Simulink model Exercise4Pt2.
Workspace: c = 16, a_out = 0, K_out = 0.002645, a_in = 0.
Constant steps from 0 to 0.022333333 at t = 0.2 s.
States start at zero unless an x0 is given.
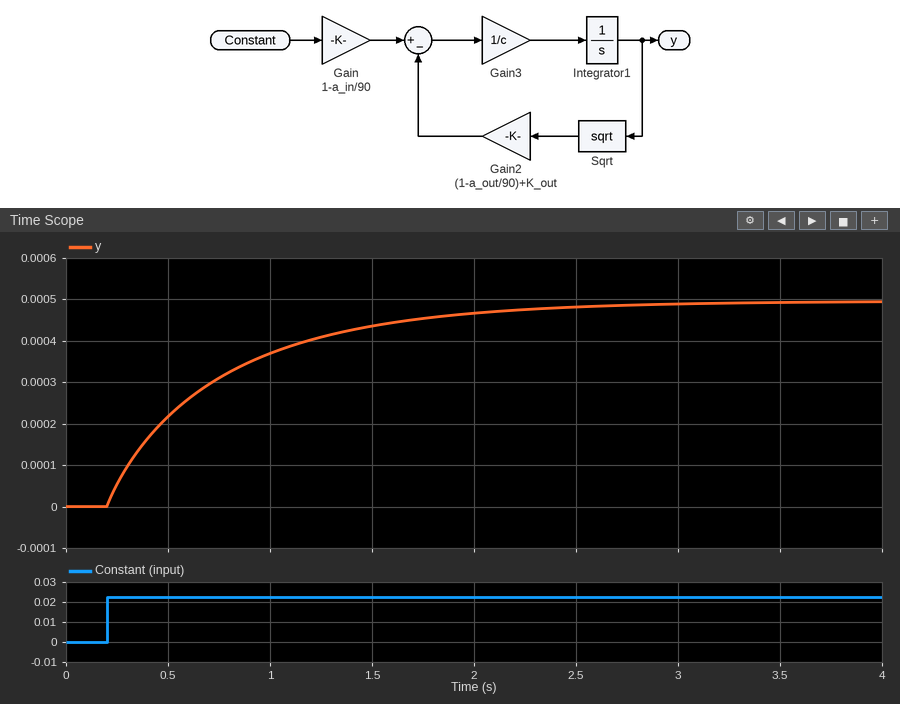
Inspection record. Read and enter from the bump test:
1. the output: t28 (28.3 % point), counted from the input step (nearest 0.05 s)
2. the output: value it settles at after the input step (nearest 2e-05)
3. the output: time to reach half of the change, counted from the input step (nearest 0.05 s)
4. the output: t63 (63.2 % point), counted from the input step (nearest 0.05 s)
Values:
0.15 s
0.00050
0.35 s
0.55 s
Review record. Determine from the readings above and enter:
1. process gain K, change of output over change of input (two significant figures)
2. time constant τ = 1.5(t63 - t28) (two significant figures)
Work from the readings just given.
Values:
0.022
0.60 s
